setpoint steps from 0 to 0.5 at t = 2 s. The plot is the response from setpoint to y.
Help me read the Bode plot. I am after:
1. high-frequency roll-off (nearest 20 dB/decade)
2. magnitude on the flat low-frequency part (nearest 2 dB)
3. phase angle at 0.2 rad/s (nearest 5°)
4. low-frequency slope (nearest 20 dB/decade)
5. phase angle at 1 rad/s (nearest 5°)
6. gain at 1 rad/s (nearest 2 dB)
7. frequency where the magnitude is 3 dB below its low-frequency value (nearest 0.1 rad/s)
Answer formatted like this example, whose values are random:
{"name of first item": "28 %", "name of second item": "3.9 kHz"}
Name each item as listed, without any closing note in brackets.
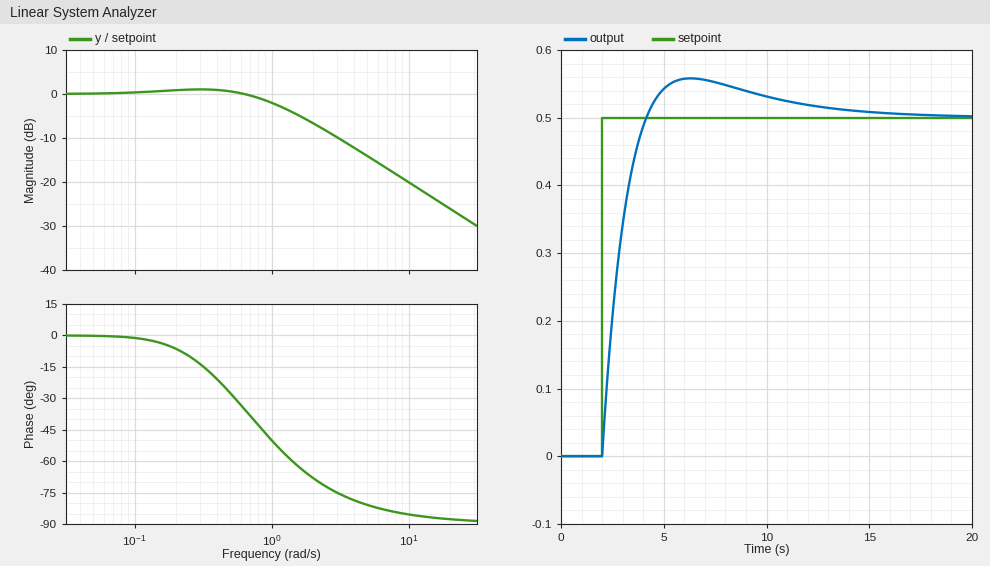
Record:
{"high-frequency roll-off": "-20 dB/decade", "magnitude on the flat low-frequency part": "0 dB", "phase angle at 0.2 rad/s": "-5°", "low-frequency slope": "0 dB/decade", "phase angle at 1 rad/s": "-50°", "gain at 1 rad/s": "-2 dB", "frequency where the magnitude is 3 dB below its low-frequency value": "1.2 rad/s"}
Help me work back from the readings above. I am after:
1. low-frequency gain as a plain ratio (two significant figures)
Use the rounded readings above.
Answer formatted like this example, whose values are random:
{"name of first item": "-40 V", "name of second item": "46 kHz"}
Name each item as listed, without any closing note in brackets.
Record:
{"low-frequency gain as a plain ratio": "1.0"}
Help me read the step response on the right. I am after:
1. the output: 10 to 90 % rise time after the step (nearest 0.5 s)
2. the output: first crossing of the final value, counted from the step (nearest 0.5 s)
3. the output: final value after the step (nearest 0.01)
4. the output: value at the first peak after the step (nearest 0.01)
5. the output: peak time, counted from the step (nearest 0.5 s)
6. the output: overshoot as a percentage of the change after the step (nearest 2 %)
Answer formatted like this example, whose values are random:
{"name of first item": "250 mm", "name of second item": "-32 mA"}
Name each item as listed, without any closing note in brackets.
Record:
{"the output: 10 to 90 % rise time after the step": "1.5 s", "the output: first crossing of the final value, counted from the step": "2.0 s", "the output: final value after the step": "0.50", "the output: value at the first peak after the step": "0.56", "the output: peak time, counted from the step": "4.5 s", "the output: overshoot as a percentage of the change after the step": "12 %"}
